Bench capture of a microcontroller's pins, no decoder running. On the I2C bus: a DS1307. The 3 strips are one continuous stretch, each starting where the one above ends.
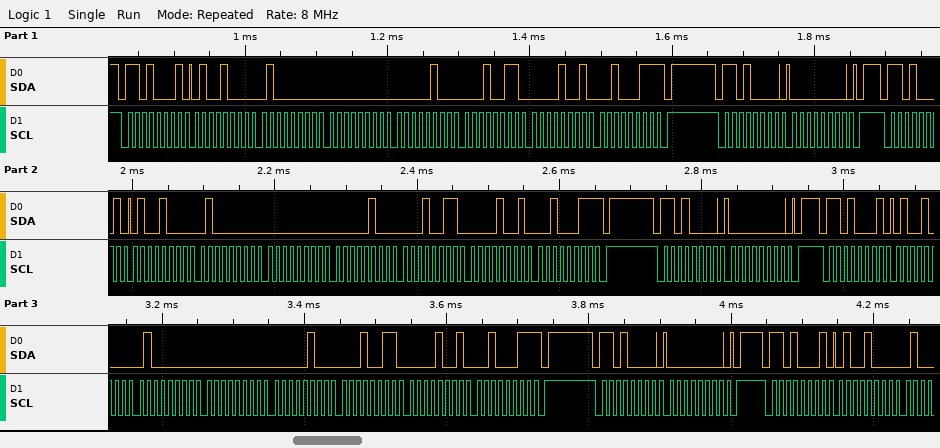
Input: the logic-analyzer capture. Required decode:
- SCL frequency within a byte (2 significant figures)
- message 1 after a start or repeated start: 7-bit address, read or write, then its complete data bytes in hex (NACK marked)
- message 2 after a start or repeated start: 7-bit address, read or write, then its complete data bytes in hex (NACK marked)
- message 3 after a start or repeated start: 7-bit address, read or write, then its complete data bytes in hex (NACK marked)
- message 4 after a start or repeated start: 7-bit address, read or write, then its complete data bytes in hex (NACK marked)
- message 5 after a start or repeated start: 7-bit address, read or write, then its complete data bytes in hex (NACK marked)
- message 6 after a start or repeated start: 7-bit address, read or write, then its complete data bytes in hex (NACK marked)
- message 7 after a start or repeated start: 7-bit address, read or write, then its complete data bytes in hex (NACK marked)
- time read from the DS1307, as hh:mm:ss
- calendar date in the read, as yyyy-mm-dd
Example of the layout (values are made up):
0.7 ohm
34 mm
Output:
100 kHz
0x68 read: 48 40 00 04 13 09 23 NACK
0x68 write: 00
0x68 read: 48 40 00 04 13 09 23 NACK
0x68 write: 00
0x68 read: 48 40 00 04 13 09 23 NACK
0x68 write: 00
0x68 read: 48
00:40:48
2023-09-13
